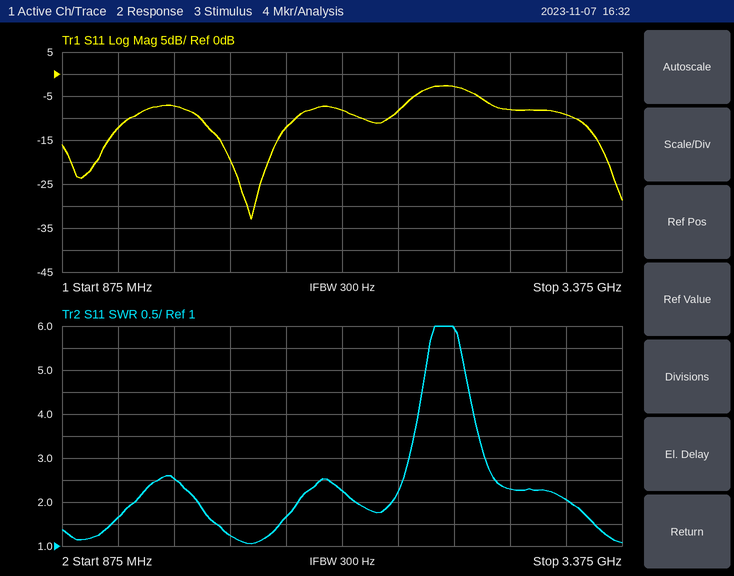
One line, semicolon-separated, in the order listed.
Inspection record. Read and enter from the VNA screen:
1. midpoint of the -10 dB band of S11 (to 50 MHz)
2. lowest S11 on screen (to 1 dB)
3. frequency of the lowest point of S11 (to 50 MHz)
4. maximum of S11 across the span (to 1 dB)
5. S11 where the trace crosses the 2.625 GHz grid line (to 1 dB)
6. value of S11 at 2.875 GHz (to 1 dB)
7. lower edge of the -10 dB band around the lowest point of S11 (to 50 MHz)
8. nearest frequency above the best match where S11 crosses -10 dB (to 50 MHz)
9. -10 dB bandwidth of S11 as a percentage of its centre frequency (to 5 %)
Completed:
1.70 GHz; -33 dB; 1.70 GHz; -3 dB; -3 dB; -8 dB; 1.50 GHz; 1.90 GHz; 25 %
